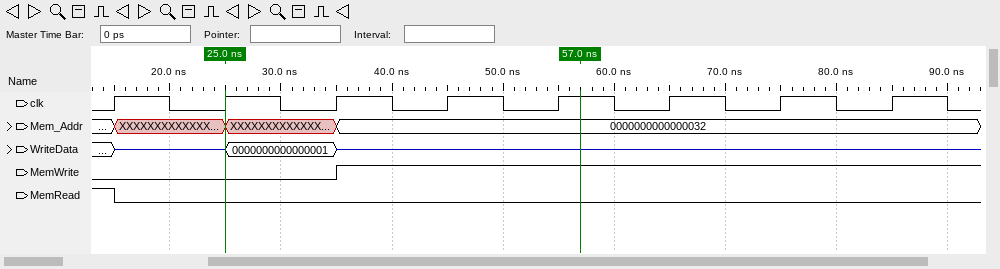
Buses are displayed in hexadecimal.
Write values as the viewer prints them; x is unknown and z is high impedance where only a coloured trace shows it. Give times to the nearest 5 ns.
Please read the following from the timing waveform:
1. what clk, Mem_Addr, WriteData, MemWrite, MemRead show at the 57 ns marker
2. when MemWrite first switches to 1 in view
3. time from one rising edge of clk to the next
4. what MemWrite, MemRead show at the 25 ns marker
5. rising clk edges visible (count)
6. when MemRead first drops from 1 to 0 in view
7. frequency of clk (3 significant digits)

clk=1, Mem_Addr=0000000000000032, WriteData=z, MemWrite=1, MemRead=0
35 ns
10 ns
MemWrite=0, MemRead=0
8
15 ns
100 MHz
